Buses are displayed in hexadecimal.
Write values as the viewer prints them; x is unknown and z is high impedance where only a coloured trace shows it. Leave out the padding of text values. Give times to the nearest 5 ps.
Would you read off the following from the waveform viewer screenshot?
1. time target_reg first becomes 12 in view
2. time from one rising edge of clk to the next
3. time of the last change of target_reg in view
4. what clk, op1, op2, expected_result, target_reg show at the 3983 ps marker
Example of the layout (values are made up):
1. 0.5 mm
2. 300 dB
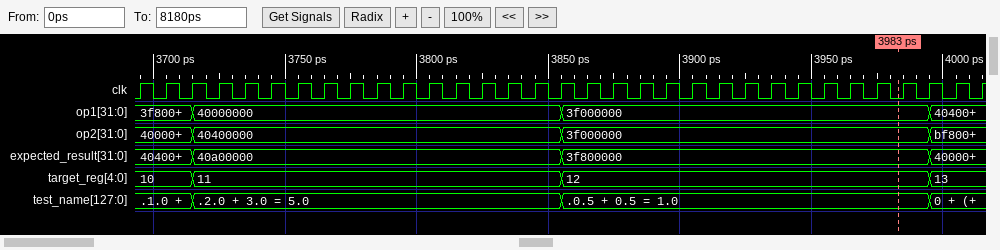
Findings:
1. 3855 ps
2. 10 ps
3. 3995 ps
4. clk=0, op1=3f000000, op2=3f000000, expected_result=3f800000, target_reg=12
